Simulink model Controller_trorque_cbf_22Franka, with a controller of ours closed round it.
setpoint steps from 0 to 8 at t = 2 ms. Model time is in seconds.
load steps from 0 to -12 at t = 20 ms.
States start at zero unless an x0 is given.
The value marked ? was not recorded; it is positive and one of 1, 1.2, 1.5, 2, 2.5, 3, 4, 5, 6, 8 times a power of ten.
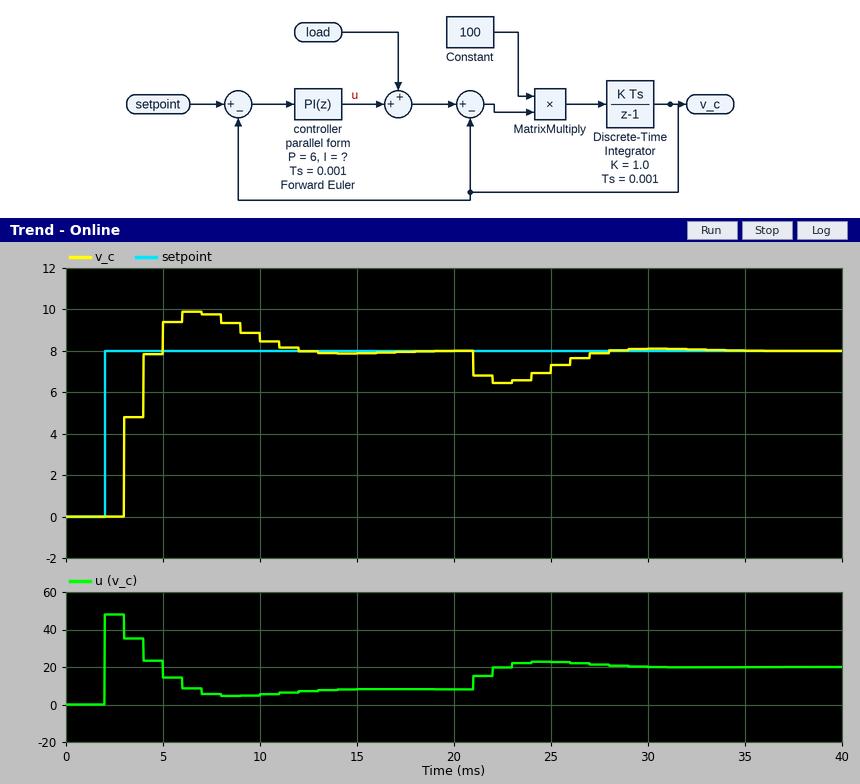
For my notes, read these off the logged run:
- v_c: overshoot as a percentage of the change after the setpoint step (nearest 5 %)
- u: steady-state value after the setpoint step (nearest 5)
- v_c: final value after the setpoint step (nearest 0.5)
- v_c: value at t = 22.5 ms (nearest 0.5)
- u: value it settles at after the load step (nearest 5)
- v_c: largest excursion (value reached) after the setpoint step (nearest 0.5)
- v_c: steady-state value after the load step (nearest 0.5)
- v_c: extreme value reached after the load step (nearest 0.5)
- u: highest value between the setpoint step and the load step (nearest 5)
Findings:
25 %
10
8.0
6.5
20
10.0
8.0
6.5
50
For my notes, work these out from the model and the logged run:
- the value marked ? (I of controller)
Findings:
2000
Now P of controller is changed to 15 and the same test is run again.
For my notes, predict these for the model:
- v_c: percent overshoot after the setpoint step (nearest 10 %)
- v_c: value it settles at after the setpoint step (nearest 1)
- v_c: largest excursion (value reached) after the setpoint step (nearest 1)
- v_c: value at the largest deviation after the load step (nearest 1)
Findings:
50 %
8
12
7
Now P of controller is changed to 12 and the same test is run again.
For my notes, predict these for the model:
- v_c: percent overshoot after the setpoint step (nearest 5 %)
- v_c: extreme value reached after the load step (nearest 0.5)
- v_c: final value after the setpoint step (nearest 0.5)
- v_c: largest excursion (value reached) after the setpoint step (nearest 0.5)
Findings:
20 %
7.0
8.0
9.5
